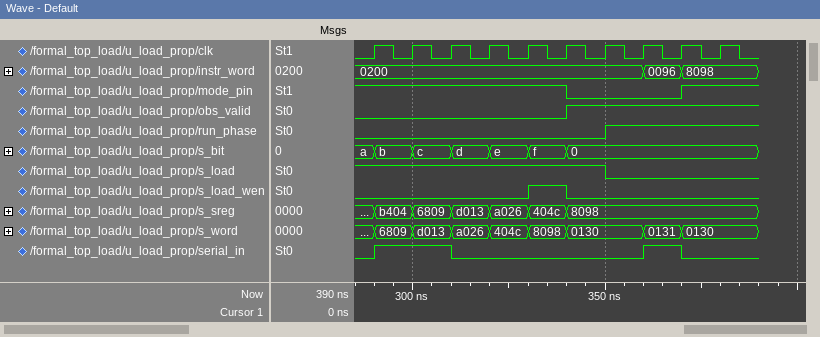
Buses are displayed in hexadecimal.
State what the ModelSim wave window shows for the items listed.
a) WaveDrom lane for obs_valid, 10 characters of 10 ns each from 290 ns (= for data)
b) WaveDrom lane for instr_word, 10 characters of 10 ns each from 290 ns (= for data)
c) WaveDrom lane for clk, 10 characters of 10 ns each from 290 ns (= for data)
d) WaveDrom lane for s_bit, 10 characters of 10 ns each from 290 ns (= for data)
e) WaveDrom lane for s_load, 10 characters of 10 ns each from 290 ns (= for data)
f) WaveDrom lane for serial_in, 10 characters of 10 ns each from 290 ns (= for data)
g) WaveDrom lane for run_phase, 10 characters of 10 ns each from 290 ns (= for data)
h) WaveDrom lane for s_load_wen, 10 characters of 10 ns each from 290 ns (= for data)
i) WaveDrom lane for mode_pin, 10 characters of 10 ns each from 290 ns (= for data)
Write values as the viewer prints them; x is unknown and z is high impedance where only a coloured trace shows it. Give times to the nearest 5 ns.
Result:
{name: 'obs_valid', wave: '0....1....'}
{name: 'instr_word', wave: '=......==.', data: '0200 0096 8098'}
{name: 'clk', wave: 'p.........'}
{name: 's_bit', wave: '======....', data: 'b c d e f 0'}
{name: 's_load', wave: '1.....0...'}
{name: 'serial_in', wave: '1.0....10.'}
{name: 'run_phase', wave: '0.....1...'}
{name: 's_load_wen', wave: '0...10....'}
{name: 'mode_pin', wave: '1....0..1.'}
